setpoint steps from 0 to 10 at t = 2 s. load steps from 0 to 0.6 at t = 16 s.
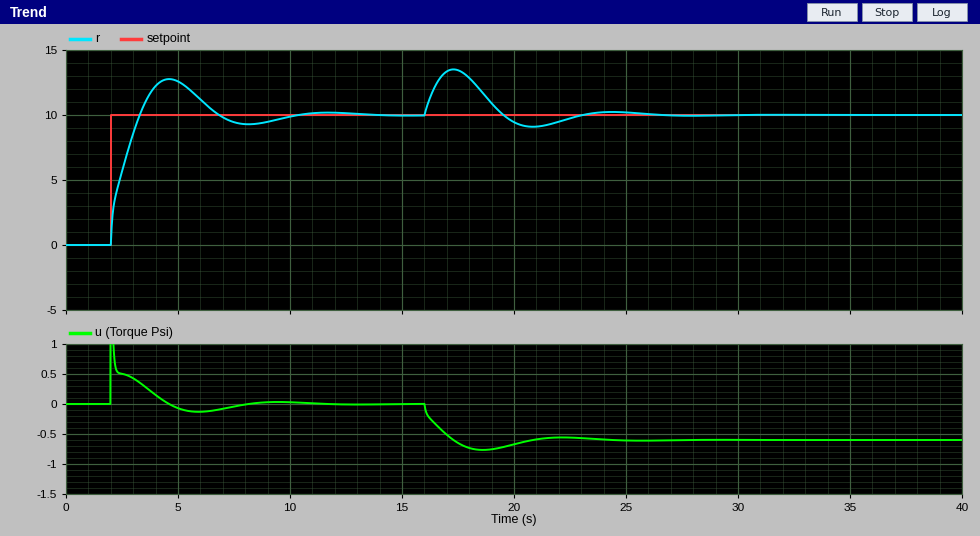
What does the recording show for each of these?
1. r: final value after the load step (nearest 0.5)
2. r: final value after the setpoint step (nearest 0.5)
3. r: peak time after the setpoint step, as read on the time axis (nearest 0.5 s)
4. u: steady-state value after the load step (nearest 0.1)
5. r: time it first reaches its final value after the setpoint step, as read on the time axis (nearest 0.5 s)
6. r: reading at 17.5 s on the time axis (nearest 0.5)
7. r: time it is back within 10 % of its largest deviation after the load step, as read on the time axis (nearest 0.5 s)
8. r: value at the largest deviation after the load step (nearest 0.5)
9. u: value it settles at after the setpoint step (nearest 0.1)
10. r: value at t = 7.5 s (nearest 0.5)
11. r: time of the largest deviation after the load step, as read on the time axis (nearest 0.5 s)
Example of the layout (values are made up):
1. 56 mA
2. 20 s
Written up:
1. 10.0
2. 10.0
3. 4.5 s
4. -0.6
5. 3.5 s
6. 13.5
7. 22.5 s
8. 13.5
9. 0.0
10. 9.5
11. 17.5 s
